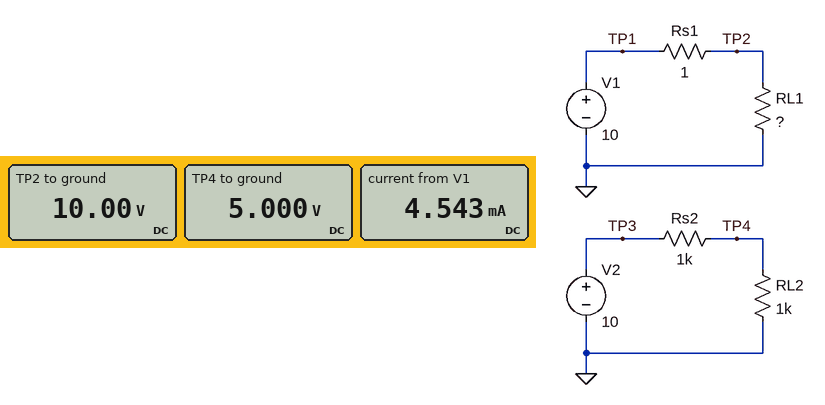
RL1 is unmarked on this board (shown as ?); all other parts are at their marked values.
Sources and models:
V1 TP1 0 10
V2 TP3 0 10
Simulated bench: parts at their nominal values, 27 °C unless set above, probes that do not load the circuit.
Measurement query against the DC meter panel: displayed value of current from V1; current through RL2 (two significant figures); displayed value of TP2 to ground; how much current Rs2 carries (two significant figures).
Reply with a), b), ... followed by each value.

a) 4.543 mA
b) 5.0 mA
c) 10.00 V
d) 5.0 mA
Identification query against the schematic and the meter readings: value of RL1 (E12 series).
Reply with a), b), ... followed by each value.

a) 2.2 kΩ
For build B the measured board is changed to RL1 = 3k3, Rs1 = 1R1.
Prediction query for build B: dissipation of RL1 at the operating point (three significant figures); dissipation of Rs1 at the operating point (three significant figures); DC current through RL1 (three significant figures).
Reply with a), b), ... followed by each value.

a) 30.3 mW
b) 10.1 µW
c) 3.03 mA
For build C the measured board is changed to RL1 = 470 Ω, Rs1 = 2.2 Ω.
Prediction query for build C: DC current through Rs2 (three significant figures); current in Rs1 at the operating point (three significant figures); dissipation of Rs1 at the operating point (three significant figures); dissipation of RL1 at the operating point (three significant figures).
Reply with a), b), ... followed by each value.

a) 5.00 mA
b) 21.2 mA
c) 987 µW
d) 211 mW
